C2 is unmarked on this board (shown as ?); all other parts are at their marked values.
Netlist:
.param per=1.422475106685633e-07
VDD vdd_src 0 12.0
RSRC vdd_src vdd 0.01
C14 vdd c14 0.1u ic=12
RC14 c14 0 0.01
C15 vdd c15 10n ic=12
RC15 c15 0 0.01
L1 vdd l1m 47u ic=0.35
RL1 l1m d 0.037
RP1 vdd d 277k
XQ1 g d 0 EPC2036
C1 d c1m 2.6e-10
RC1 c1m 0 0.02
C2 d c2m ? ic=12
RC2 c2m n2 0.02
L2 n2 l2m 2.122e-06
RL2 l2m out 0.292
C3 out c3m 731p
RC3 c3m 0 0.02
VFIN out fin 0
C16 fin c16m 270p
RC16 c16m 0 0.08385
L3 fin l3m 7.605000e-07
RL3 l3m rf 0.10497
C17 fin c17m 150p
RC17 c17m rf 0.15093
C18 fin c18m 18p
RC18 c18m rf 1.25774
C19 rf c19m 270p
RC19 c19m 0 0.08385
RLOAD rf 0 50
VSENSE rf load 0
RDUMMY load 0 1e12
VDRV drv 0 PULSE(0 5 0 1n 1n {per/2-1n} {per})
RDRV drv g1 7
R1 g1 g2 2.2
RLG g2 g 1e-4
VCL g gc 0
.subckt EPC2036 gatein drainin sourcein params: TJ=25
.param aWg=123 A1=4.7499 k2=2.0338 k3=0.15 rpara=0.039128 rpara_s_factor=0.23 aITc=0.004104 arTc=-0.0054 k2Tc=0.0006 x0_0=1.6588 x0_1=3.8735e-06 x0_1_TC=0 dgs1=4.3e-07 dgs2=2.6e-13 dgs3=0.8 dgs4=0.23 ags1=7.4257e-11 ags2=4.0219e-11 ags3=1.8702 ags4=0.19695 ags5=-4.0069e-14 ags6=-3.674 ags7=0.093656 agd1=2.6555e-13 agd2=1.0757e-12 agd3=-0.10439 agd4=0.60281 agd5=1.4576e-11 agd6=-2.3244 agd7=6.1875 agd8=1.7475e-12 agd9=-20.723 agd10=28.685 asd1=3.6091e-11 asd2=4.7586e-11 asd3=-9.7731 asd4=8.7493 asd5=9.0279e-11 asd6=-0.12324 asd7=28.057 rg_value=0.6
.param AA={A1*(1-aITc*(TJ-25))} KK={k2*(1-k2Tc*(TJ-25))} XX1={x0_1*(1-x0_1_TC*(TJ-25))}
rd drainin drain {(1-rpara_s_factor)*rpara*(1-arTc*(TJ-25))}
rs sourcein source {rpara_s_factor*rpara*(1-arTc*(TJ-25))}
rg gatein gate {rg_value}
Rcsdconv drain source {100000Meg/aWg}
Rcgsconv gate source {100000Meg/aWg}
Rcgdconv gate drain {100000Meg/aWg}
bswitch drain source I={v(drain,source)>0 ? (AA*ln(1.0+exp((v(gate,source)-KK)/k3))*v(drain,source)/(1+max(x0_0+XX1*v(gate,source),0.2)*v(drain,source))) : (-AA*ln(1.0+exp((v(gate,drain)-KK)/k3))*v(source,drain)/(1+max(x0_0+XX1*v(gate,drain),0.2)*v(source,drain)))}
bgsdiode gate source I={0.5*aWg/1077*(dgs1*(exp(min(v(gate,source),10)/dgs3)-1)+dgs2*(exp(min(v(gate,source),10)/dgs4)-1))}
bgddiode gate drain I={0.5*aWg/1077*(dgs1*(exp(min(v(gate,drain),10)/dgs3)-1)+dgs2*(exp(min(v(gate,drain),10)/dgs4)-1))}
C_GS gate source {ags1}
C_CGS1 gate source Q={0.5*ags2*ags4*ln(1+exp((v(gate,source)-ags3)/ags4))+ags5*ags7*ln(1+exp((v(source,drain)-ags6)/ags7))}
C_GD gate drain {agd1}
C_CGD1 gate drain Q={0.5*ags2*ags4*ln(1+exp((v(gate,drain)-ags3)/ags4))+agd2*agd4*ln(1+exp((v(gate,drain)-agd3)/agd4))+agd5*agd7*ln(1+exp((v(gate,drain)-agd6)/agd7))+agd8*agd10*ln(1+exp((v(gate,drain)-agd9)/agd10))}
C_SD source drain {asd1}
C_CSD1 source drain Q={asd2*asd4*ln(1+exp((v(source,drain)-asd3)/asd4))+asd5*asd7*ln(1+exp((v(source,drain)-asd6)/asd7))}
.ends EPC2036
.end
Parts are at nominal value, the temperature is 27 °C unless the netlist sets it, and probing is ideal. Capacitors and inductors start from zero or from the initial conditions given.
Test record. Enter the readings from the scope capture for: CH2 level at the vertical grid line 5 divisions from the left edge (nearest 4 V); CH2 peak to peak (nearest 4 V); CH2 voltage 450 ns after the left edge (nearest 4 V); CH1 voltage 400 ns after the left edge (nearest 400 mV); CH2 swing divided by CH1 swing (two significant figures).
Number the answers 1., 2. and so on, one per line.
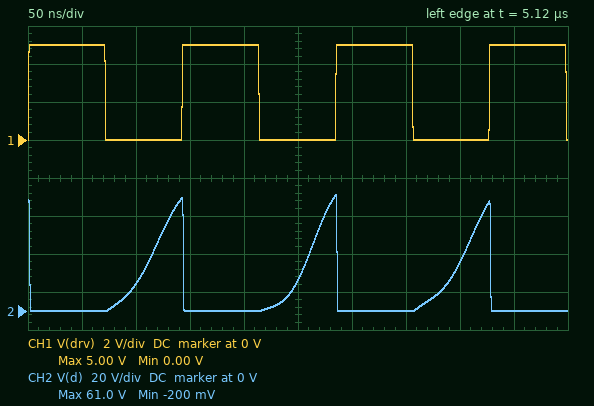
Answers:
1. 16 V
2. 60 V
3. 0 V
4. 0 V
5. 12
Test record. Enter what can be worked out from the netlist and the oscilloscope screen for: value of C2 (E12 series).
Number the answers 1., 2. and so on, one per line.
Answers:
1. 120 pF
